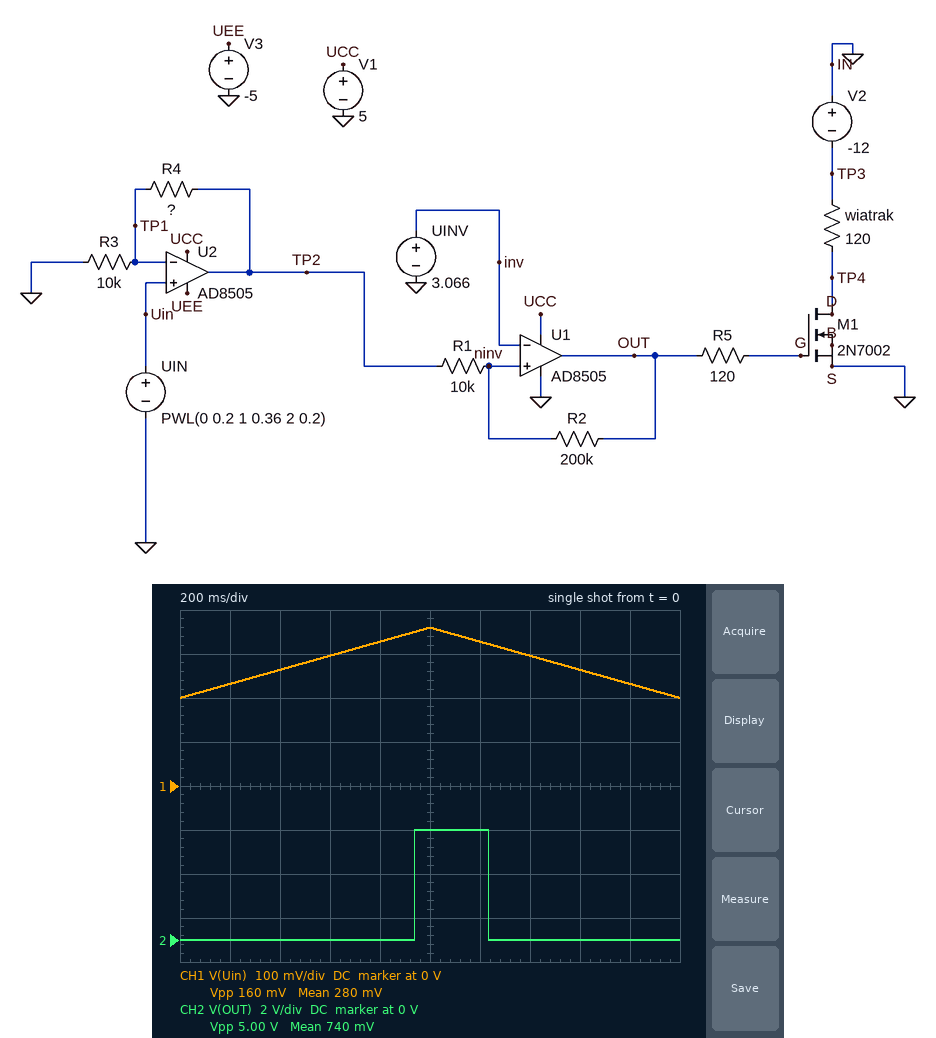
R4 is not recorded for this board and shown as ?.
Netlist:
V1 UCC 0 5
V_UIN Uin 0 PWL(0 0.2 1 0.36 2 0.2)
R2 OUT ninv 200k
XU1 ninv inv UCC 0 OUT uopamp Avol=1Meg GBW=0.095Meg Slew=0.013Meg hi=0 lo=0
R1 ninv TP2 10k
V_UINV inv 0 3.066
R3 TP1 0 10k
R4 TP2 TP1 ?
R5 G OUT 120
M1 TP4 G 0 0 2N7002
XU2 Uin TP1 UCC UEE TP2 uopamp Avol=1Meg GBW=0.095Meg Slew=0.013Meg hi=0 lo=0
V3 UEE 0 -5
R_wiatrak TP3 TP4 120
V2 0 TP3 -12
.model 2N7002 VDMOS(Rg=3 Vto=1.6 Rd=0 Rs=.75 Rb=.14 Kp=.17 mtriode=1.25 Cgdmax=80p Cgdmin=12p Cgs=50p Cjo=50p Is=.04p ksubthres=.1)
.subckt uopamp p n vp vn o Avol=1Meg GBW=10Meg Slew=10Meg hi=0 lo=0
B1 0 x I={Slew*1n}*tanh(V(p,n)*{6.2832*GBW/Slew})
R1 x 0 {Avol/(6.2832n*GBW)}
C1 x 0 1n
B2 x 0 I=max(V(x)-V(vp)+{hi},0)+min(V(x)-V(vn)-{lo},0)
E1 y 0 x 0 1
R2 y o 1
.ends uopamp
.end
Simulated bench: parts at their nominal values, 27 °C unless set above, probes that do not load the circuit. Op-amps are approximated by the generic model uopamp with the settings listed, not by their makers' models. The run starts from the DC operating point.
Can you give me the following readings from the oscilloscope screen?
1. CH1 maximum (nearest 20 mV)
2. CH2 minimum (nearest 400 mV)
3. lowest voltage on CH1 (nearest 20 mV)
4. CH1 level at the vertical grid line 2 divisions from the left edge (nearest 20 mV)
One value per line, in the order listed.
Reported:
360 mV
0 V
200 mV
260 mV
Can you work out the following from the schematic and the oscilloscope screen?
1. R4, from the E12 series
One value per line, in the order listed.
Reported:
82 kΩ
